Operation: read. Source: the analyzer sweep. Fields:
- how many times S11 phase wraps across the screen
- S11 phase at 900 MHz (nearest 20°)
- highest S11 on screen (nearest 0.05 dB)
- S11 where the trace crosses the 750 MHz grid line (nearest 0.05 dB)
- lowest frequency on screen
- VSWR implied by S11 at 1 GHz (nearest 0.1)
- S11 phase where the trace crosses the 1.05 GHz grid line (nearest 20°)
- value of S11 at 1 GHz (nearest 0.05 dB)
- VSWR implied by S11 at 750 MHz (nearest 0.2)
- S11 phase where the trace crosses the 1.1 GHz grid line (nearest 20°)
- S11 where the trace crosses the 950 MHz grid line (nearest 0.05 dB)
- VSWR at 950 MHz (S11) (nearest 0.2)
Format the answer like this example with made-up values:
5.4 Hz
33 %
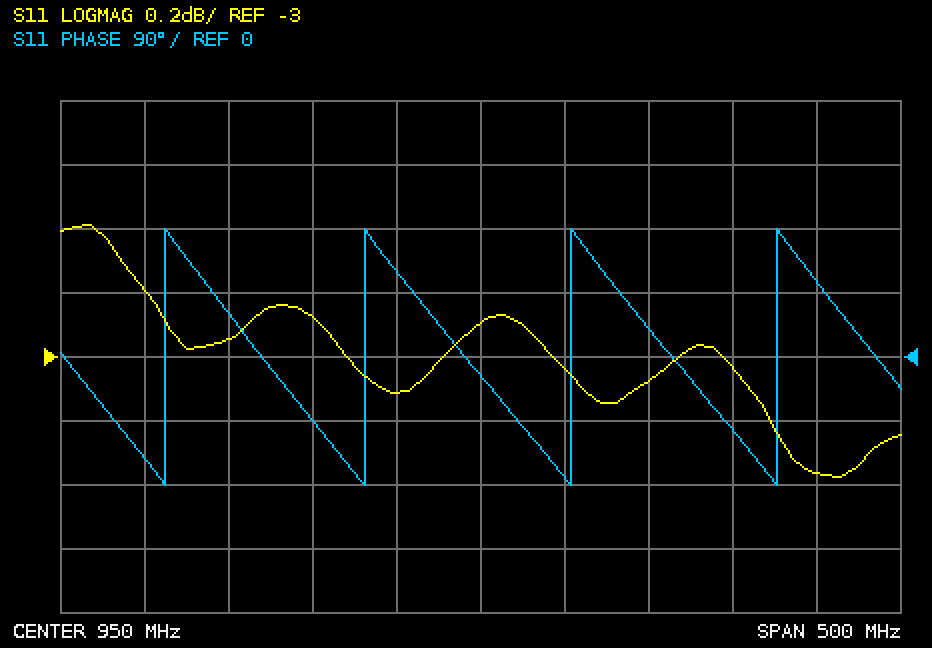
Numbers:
4
120°
-2.60 dB
-2.80 dB
700 MHz
5.8
40°
-3.05 dB
6.2
-100°
-2.90 dB
6.0
